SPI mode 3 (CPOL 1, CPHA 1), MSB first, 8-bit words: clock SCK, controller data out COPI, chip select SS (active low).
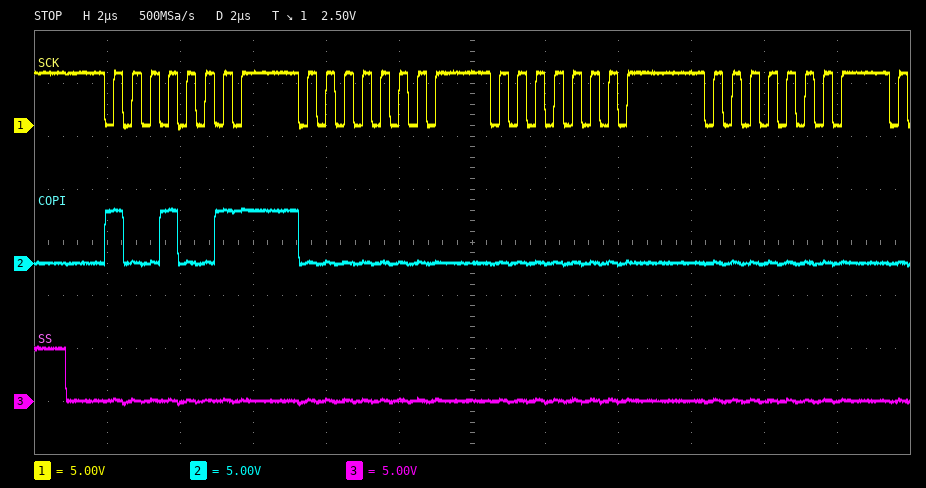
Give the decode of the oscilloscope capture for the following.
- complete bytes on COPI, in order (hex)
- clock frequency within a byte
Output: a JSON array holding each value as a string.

["93 00 00 00", "2 MHz"]
